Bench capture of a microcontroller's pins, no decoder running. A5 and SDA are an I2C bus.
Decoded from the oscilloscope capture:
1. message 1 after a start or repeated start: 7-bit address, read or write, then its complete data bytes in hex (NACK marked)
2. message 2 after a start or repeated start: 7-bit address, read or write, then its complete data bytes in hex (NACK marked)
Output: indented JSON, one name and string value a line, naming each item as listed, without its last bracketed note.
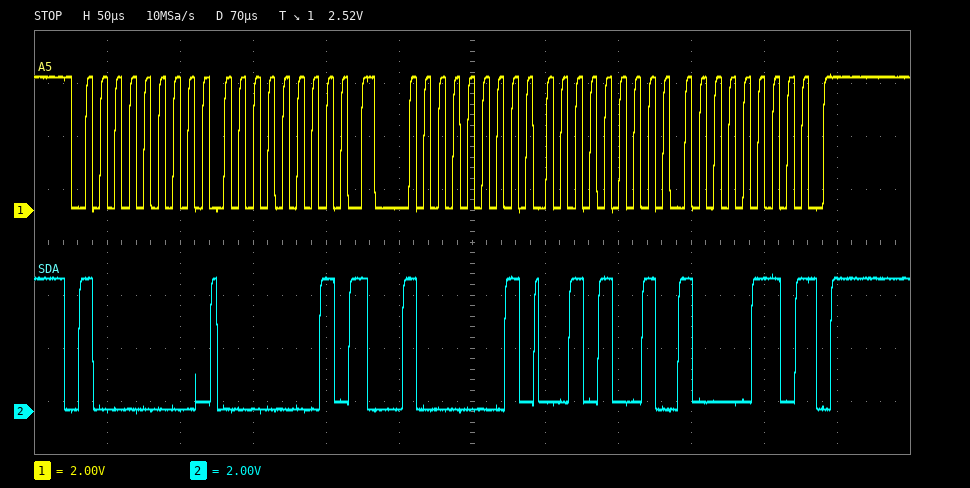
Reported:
{
  "message 1 after a start or repeated start: 7-bit address, read or write, then its complete data bytes in hex": "0x40 write: 01",
  "message 2 after a start or repeated start: 7-bit address, read or write, then its complete data bytes in hex": "0x40 read: 29 86 NACK"
}
